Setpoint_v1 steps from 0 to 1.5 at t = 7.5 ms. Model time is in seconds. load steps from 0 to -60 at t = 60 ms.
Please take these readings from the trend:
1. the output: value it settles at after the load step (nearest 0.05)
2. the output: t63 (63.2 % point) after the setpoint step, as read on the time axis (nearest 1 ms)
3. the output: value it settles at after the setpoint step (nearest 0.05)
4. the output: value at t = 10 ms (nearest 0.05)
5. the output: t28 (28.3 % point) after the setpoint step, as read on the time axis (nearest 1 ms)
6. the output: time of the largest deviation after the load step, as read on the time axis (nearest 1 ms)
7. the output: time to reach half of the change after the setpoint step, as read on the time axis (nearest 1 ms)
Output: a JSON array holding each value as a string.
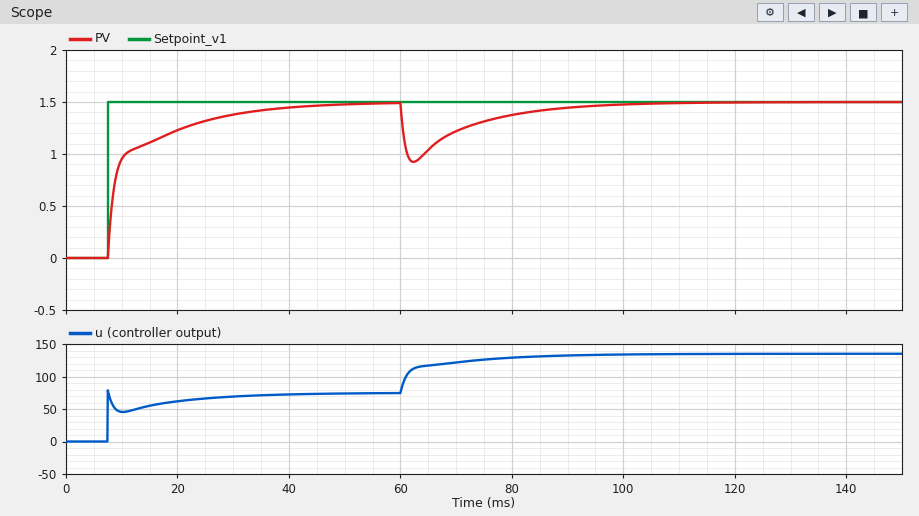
["1.50", "10 ms", "1.50", "0.95", "8 ms", "62 ms", "9 ms"]
